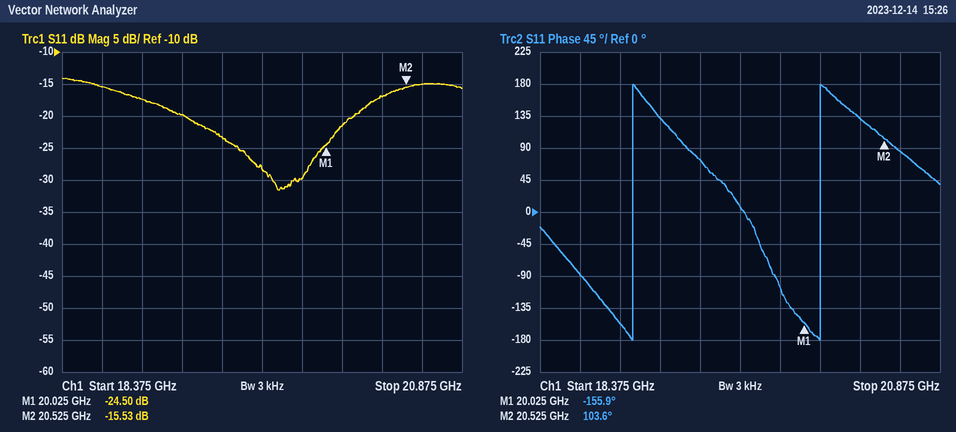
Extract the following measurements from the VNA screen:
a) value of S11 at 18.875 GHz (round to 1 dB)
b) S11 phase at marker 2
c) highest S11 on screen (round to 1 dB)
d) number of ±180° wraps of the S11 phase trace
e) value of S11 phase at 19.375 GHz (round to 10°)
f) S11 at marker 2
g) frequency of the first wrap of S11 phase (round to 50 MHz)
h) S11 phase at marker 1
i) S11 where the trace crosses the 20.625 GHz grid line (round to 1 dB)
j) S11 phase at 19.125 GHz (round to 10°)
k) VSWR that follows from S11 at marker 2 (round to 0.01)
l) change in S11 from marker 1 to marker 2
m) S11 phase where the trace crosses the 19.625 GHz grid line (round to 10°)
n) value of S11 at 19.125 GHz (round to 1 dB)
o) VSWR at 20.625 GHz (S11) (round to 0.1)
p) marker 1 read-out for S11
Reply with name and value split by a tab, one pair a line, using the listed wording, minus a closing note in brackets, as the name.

value of S11 at 18.875 GHz	-17 dB
S11 phase at marker 2	103.6°
highest S11 on screen	-14 dB
number of ±180° wraps of the S11 phase trace	2
value of S11 phase at 19.375 GHz	70°
S11 at marker 2	-15.53 dB
frequency of the first wrap of S11 phase	18.95 GHz
S11 phase at marker 1	-155.9°
S11 where the trace crosses the 20.625 GHz grid line	-15 dB
S11 phase at 19.125 GHz	130°
VSWR that follows from S11 at marker 2	1.40
change in S11 from marker 1 to marker 2	8.97 dB
S11 phase where the trace crosses the 19.625 GHz grid line	10°
value of S11 at 19.125 GHz	-20 dB
VSWR at 20.625 GHz (S11)	1.4
marker 1 read-out for S11	-24.50 dB
